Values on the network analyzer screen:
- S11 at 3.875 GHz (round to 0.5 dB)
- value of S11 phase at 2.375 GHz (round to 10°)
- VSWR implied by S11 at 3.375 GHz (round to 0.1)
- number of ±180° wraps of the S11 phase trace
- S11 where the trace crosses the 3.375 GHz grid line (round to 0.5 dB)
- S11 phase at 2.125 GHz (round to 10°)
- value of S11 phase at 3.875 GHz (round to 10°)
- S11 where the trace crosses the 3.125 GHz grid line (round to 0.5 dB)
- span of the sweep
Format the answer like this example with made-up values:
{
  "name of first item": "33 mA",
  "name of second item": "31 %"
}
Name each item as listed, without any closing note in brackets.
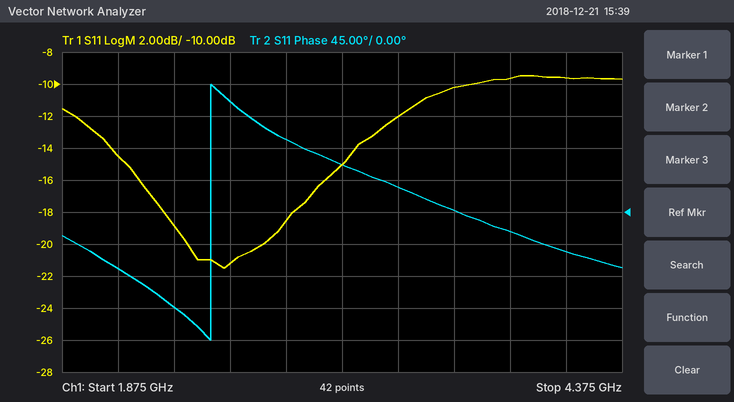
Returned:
{
  "S11 at 3.875 GHz": "-9.5 dB",
  "value of S11 phase at 2.375 GHz": "-130°",
  "VSWR implied by S11 at 3.375 GHz": "1.7",
  "number of ±180° wraps of the S11 phase trace": "1",
  "S11 where the trace crosses the 3.375 GHz grid line": "-12.0 dB",
  "S11 phase at 2.125 GHz": "-80°",
  "value of S11 phase at 3.875 GHz": "-30°",
  "S11 where the trace crosses the 3.125 GHz grid line": "-15.0 dB",
  "span of the sweep": "2.5 GHz"
}
